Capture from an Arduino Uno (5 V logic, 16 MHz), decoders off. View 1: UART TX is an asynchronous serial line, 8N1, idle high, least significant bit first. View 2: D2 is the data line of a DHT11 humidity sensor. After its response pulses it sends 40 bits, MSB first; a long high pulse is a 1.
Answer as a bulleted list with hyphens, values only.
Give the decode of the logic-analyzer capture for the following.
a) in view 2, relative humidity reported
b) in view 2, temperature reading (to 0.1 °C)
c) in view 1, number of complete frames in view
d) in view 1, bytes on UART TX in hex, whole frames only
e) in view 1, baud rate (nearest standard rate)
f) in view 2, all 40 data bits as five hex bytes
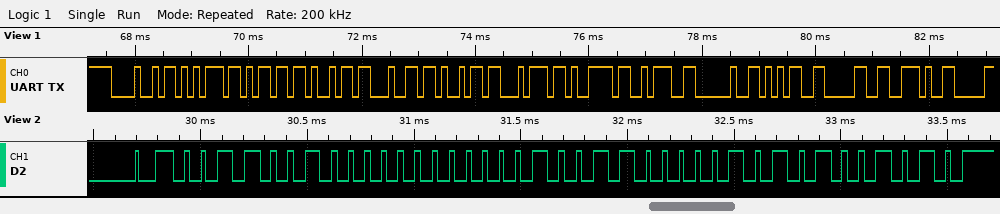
- 50 %
- 19.5 °C
- 13
- 48 75 6D 69 64 69 74 79 3A 20 35 30 2E
- 9600 baud
- 32 00 13 05 4A
